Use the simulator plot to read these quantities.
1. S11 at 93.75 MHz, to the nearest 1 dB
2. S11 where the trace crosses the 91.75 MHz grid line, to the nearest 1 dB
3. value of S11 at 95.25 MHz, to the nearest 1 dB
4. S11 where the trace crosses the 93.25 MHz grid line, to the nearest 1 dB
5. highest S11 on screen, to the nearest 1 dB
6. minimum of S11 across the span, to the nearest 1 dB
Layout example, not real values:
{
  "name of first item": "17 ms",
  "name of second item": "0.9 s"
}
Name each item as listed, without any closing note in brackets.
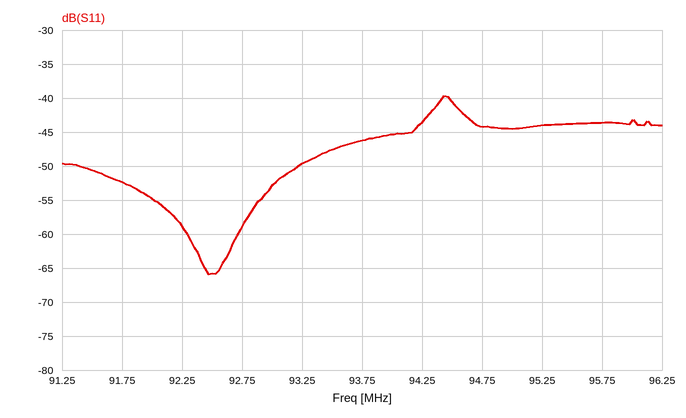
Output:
{
  "S11 at 93.75 MHz, to the nearest 1 dB": "-46 dB",
  "S11 where the trace crosses the 91.75 MHz grid line, to the nearest 1 dB": "-52 dB",
  "value of S11 at 95.25 MHz, to the nearest 1 dB": "-44 dB",
  "S11 where the trace crosses the 93.25 MHz grid line, to the nearest 1 dB": "-50 dB",
  "highest S11 on screen, to the nearest 1 dB": "-40 dB",
  "minimum of S11 across the span, to the nearest 1 dB": "-66 dB"
}
